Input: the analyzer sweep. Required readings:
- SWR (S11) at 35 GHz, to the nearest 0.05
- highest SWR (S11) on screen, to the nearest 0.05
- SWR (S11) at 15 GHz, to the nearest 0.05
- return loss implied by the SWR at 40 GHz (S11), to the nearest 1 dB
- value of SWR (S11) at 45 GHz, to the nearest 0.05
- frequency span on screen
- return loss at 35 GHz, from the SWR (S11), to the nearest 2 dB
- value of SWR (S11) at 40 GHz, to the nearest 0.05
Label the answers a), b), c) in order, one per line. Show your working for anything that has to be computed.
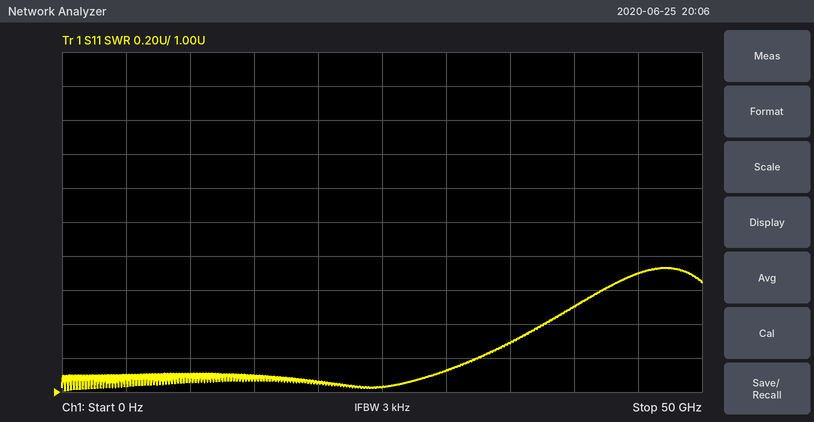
a) 1.30
b) 1.75
c) 1.10
d) −20 log10((1.5 − 1)/(1.5 + 1)) ≈ 14 dB
e) 1.70
f) 50 GHz
g) −20 log10((1.3 − 1)/(1.3 + 1)) ≈ 18 dB
h) 1.50
